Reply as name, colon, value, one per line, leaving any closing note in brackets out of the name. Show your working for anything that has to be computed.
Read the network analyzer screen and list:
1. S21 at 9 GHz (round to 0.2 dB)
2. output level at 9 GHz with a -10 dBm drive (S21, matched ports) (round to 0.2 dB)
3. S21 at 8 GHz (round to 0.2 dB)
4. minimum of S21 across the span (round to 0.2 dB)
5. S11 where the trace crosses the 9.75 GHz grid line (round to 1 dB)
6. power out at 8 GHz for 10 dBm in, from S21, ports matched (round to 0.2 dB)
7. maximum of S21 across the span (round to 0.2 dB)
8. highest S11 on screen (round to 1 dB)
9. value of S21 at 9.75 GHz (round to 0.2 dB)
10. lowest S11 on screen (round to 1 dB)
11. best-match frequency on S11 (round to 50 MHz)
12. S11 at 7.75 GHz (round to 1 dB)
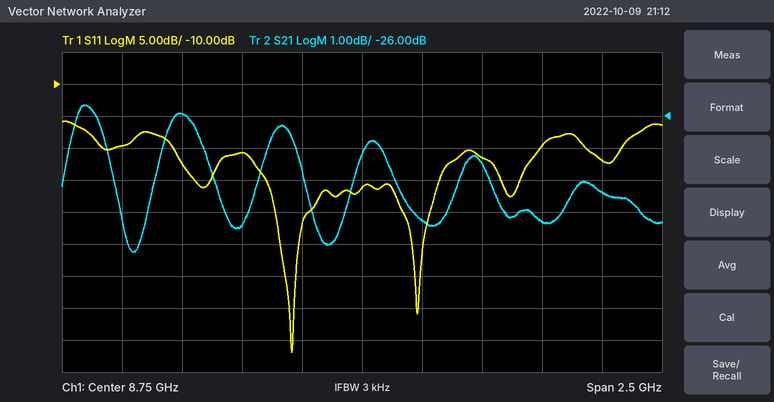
S21 at 9 GHz: -29.2 dB
output level at 9 GHz with a -10 dBm drive (S21, matched ports): -10 dBm + (-29.2 dB) = -39.2 dBm
S21 at 8 GHz: -26.0 dB
minimum of S21 across the span: -30.2 dB
S11 where the trace crosses the 9.75 GHz grid line: -22 dB
power out at 8 GHz for 10 dBm in, from S21, ports matched: 10 dBm + (-26.0 dB) = -16.0 dBm
maximum of S21 across the span: -25.6 dB
highest S11 on screen: -16 dB
value of S21 at 9.75 GHz: -28.4 dB
lowest S11 on screen: -52 dB
best-match frequency on S11: 8.45 GHz
S11 at 7.75 GHz: -20 dB
